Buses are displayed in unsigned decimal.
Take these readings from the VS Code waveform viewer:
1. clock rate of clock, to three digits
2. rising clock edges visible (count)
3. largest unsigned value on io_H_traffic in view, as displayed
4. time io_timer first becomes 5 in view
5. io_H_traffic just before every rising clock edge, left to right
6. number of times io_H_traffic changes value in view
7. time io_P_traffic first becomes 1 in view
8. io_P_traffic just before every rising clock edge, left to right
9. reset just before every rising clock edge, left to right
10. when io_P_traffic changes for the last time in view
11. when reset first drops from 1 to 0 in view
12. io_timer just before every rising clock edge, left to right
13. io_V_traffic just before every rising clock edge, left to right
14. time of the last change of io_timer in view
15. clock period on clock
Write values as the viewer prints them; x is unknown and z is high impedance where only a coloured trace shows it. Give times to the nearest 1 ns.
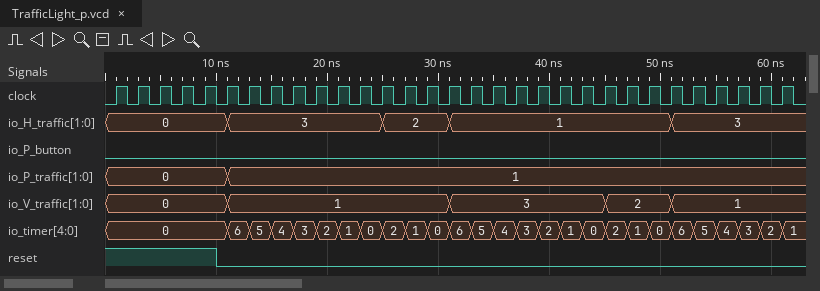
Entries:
500 MHz
31
3
13 ns
0, 0, 0, 0, 0, 0, 3, 3, 3, 3, 3, 3, 3, 2, 2, 2, 1, 1, 1, 1, 1, 1, 1, 1, 1, 1, 3, 3, 3, 3, 3
4
11 ns
0, 0, 0, 0, 0, 0, 1, 1, 1, 1, 1, 1, 1, 1, 1, 1, 1, 1, 1, 1, 1, 1, 1, 1, 1, 1, 1, 1, 1, 1, 1
1 1 1 1 1 0 0 0 0 0 0 0 0 0 0 0 0 0 0 0 0 0 0 0 0 0 0 0 0 0 0
11 ns
10 ns
0, 0, 0, 0, 0, 0, 6, 5, 4, 3, 2, 1, 0, 2, 1, 0, 6, 5, 4, 3, 2, 1, 0, 2, 1, 0, 6, 5, 4, 3, 2
0, 0, 0, 0, 0, 0, 1, 1, 1, 1, 1, 1, 1, 1, 1, 1, 3, 3, 3, 3, 3, 3, 3, 2, 2, 2, 1, 1, 1, 1, 1
61 ns
2 ns
